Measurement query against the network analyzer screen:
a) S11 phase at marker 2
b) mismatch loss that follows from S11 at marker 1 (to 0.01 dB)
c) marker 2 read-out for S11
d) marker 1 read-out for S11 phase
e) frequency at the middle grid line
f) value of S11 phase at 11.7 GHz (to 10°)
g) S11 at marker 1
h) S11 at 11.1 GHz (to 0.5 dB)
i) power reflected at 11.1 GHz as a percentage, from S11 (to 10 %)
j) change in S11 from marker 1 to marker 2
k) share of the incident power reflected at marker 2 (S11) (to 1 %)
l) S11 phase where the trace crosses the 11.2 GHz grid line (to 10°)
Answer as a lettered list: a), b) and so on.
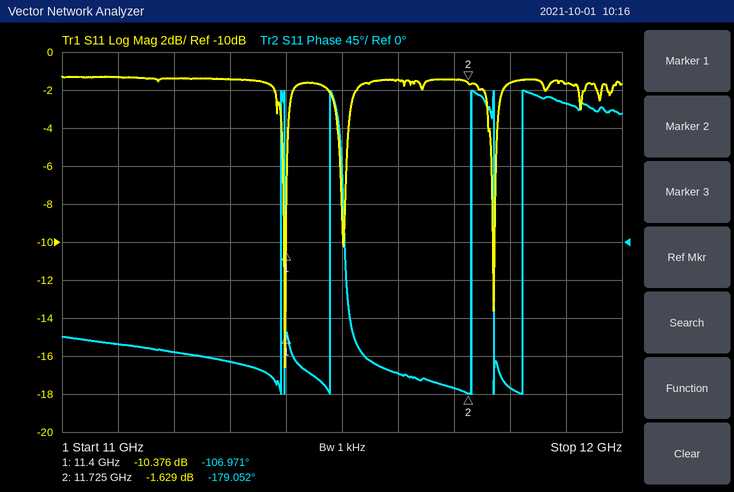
a) -179.052°
b) 0.42 dB
c) -1.629 dB
d) -106.971°
e) 11.5 GHz
f) -170°
g) -10.376 dB
h) -1.5 dB
i) 70 %
j) 8.747 dB
k) 69 %
l) -130°
